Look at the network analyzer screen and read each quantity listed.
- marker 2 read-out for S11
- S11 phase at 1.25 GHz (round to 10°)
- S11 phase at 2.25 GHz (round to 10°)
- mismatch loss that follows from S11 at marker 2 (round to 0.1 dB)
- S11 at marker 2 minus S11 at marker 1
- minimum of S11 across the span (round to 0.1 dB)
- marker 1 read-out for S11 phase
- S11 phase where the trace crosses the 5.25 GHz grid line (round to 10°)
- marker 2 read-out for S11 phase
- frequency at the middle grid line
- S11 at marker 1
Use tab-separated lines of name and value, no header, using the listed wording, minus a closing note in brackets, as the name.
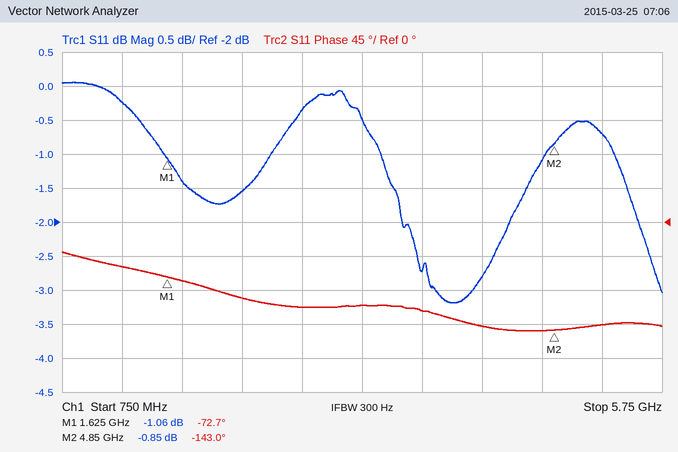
marker 2 read-out for S11	-0.85 dB
S11 phase at 1.25 GHz	-60°
S11 phase at 2.25 GHz	-100°
mismatch loss that follows from S11 at marker 2	7.5 dB
S11 at marker 2 minus S11 at marker 1	0.21 dB
minimum of S11 across the span	-3.2 dB
marker 1 read-out for S11 phase	-72.7°
S11 phase where the trace crosses the 5.25 GHz grid line	-140°
marker 2 read-out for S11 phase	-143.0°
frequency at the middle grid line	3.25 GHz
S11 at marker 1	-1.06 dB
